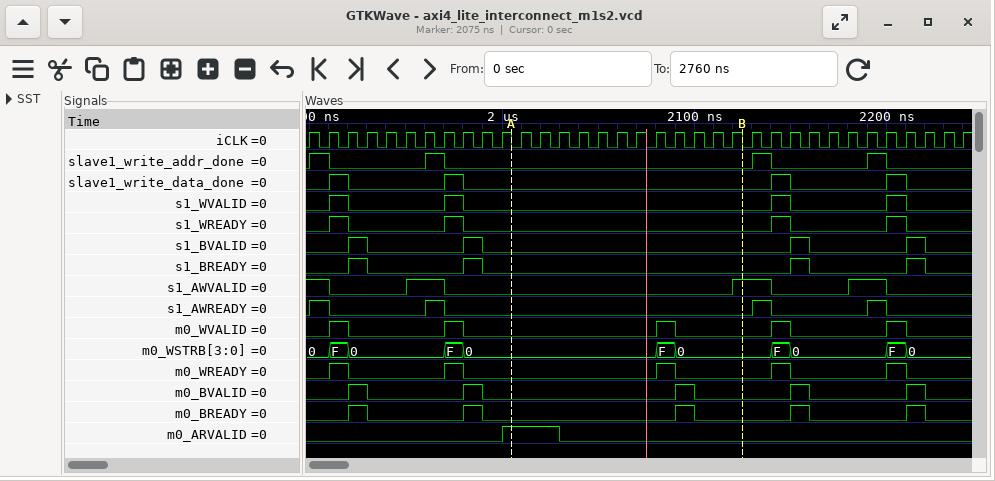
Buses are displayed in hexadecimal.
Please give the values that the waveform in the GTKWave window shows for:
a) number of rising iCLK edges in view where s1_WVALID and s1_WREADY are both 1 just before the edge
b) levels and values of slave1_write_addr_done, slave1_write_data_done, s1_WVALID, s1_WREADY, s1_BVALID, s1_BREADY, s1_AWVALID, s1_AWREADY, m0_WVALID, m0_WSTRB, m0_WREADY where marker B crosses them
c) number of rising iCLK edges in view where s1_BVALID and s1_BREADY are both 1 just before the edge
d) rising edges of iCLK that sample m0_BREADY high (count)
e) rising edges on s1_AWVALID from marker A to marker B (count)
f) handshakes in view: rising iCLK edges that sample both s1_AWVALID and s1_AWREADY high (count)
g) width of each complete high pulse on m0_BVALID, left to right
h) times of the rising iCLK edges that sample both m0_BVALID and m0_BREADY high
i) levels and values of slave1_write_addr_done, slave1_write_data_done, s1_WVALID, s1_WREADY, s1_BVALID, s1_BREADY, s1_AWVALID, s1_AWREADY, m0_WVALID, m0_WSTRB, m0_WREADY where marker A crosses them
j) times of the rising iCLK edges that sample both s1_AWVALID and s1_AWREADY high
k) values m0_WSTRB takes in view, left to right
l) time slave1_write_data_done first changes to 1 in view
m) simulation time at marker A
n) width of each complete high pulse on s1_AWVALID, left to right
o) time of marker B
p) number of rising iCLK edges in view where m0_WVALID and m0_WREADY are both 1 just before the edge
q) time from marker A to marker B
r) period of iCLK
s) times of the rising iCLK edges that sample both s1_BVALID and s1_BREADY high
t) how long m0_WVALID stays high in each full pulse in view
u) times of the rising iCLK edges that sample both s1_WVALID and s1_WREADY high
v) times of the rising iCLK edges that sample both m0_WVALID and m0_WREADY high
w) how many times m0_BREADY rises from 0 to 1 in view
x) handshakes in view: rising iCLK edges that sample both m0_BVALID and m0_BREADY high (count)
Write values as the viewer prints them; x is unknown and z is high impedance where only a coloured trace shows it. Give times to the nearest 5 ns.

4
slave1_write_addr_done=0, slave1_write_data_done=0, s1_WVALID=0, s1_WREADY=0, s1_BVALID=0, s1_BREADY=0, s1_AWVALID=1, s1_AWREADY=0, m0_WVALID=0, m0_WSTRB=0, m0_WREADY=0
4
5
1
4
10 ns, 10 ns, 10 ns, 10 ns, 10 ns
1930 ns, 1990 ns, 2100 ns, 2160 ns, 2220 ns
slave1_write_addr_done=0, slave1_write_data_done=0, s1_WVALID=0, s1_WREADY=0, s1_BVALID=0, s1_BREADY=0, s1_AWVALID=0, s1_AWREADY=0, m0_WVALID=0, m0_WSTRB=0, m0_WREADY=0
1910 ns, 1970 ns, 2140 ns, 2200 ns
0, F, 0, F, 0, F, 0, F, 0, F, 0
1910 ns
2005 ns
20 ns, 20 ns, 20 ns
2125 ns
5
120 ns
10 ns
1930 ns, 1990 ns, 2160 ns, 2220 ns
10 ns, 10 ns, 10 ns, 10 ns, 10 ns
1920 ns, 1980 ns, 2150 ns, 2210 ns
1920 ns, 1980 ns, 2090 ns, 2150 ns, 2210 ns
5
5
